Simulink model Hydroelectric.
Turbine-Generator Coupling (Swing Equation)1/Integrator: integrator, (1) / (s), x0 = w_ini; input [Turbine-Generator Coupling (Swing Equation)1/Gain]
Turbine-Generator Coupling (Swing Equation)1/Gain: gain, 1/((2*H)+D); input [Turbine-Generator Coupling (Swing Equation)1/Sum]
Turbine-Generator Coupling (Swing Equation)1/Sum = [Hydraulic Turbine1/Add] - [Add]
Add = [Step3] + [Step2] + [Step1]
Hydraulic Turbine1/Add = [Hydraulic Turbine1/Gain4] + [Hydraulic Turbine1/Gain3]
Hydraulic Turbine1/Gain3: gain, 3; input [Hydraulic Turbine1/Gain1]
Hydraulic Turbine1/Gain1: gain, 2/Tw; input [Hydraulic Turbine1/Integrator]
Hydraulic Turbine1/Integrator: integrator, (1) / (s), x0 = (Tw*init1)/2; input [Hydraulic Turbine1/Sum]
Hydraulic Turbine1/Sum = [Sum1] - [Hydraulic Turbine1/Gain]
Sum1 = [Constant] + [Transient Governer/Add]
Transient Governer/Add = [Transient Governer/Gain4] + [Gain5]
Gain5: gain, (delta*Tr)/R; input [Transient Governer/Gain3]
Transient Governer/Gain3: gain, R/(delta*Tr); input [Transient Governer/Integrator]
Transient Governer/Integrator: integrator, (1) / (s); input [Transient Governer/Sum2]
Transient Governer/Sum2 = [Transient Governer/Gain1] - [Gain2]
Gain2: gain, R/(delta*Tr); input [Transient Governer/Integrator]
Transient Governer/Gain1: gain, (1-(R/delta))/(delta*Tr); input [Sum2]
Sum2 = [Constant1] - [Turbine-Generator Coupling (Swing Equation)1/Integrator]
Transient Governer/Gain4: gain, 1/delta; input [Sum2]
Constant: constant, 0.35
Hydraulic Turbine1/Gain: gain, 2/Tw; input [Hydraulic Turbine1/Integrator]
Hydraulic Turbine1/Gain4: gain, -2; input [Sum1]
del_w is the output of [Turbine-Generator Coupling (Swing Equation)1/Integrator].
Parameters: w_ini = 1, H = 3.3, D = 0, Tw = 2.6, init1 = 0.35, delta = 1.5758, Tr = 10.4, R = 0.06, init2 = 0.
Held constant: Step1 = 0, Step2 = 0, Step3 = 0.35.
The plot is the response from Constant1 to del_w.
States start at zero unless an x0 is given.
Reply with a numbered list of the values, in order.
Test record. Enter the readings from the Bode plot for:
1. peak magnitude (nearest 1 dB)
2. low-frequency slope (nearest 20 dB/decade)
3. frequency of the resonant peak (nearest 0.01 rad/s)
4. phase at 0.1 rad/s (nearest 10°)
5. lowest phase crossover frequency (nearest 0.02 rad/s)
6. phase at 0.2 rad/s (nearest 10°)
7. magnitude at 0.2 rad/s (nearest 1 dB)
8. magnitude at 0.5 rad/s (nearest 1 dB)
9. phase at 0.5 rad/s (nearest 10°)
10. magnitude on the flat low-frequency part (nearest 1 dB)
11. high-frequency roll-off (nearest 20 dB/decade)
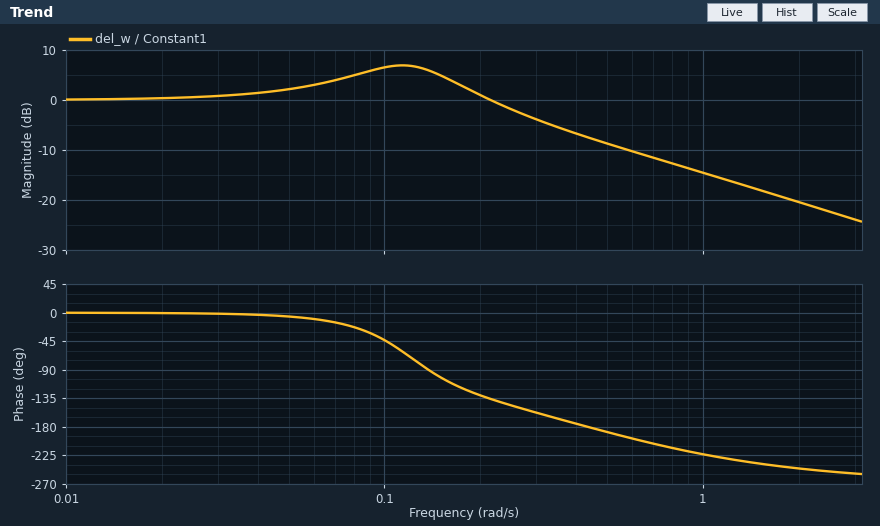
1. 7 dB
2. 0 dB/decade
3. 0.11 rad/s
4. -40°
5. 0.44 rad/s
6. -130°
7. 1 dB
8. -9 dB
9. -190°
10. 0 dB
11. -20 dB/decade
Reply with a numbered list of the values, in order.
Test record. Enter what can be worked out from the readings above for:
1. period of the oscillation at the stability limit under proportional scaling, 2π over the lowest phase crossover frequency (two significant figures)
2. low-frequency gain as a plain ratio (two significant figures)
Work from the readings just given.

1. 14 s
2. 1.0
